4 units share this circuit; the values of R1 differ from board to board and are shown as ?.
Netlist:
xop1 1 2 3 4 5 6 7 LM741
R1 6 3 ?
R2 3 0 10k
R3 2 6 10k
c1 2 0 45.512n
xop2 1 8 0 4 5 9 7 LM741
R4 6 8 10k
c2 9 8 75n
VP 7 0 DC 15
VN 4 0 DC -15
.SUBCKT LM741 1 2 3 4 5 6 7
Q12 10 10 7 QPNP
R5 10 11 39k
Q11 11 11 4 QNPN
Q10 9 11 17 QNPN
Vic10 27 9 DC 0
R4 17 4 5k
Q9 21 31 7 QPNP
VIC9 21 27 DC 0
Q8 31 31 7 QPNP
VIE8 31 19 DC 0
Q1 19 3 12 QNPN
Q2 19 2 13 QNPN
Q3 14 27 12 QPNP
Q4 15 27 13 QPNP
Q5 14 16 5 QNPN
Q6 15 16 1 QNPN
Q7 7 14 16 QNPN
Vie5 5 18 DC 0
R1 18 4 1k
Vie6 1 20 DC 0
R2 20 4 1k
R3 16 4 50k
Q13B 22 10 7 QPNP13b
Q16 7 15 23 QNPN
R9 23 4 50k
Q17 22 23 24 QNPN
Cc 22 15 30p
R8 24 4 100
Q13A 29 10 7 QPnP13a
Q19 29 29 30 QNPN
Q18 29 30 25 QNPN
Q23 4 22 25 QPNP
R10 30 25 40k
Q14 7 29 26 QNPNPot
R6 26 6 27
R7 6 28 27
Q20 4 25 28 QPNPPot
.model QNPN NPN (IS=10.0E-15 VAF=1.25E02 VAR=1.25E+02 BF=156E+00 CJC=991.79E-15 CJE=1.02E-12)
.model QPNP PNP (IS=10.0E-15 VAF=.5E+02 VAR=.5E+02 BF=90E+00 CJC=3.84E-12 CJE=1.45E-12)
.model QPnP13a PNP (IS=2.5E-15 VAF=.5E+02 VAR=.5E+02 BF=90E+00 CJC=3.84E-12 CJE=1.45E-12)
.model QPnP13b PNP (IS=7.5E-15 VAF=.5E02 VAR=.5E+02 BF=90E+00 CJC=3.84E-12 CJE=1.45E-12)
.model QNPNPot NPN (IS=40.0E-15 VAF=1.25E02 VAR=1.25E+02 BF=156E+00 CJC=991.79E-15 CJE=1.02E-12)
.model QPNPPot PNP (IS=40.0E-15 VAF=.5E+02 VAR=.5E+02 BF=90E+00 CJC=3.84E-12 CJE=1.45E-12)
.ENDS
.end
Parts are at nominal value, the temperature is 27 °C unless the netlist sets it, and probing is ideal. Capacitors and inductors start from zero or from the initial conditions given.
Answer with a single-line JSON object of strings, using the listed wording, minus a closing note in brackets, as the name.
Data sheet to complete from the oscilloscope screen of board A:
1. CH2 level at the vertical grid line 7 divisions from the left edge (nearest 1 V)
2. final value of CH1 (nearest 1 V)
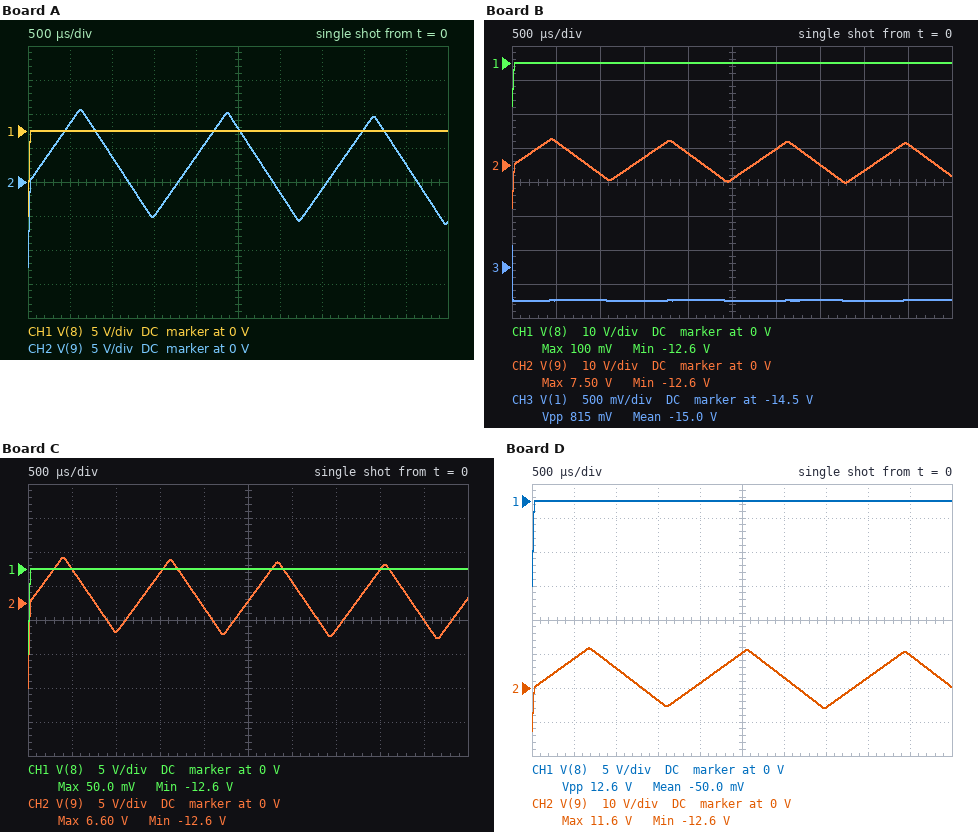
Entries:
{"CH2 level at the vertical grid line 7 divisions from the left edge": "-1 V", "final value of CH1": "0 V"}
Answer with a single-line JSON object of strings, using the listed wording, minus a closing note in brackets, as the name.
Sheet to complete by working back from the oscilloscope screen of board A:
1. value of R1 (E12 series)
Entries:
{"value of R1": "3.9 kΩ"}
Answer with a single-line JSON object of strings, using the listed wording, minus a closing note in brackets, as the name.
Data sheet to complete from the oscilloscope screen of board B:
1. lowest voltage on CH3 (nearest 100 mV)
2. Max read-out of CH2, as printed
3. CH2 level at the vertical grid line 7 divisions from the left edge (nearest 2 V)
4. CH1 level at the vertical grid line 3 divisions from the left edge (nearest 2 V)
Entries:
{"lowest voltage on CH3": "-15.0 V", "Max read-out of CH2, as printed": "7.50 V", "CH2 level at the vertical grid line 7 divisions from the left edge": "0 V", "CH1 level at the vertical grid line 3 divisions from the left edge": "0 V"}
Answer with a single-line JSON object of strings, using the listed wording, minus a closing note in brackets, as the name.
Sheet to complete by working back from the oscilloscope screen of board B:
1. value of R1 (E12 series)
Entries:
{"value of R1": "6.8 kΩ"}
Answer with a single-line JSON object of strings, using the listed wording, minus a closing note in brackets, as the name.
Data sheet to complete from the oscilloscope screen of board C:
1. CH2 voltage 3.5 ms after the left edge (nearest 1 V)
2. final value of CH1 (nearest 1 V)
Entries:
{"CH2 voltage 3.5 ms after the left edge": "-4 V", "final value of CH1": "0 V"}
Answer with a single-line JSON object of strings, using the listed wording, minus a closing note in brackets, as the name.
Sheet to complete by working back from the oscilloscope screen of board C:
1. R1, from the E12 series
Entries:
{"R1, from the E12 series": "8.2 kΩ"}
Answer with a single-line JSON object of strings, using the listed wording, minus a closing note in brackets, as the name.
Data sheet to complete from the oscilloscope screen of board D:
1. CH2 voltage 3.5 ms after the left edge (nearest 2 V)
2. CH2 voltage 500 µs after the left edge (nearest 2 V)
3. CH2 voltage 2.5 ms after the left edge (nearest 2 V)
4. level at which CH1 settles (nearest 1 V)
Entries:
{"CH2 voltage 3.5 ms after the left edge": "-6 V", "CH2 voltage 500 µs after the left edge": "8 V", "CH2 voltage 2.5 ms after the left edge": "10 V", "level at which CH1 settles": "0 V"}
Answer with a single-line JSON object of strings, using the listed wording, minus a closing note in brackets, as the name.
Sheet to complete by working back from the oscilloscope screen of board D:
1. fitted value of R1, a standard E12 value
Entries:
{"fitted value of R1, a standard E12 value": "3.3 kΩ"}
